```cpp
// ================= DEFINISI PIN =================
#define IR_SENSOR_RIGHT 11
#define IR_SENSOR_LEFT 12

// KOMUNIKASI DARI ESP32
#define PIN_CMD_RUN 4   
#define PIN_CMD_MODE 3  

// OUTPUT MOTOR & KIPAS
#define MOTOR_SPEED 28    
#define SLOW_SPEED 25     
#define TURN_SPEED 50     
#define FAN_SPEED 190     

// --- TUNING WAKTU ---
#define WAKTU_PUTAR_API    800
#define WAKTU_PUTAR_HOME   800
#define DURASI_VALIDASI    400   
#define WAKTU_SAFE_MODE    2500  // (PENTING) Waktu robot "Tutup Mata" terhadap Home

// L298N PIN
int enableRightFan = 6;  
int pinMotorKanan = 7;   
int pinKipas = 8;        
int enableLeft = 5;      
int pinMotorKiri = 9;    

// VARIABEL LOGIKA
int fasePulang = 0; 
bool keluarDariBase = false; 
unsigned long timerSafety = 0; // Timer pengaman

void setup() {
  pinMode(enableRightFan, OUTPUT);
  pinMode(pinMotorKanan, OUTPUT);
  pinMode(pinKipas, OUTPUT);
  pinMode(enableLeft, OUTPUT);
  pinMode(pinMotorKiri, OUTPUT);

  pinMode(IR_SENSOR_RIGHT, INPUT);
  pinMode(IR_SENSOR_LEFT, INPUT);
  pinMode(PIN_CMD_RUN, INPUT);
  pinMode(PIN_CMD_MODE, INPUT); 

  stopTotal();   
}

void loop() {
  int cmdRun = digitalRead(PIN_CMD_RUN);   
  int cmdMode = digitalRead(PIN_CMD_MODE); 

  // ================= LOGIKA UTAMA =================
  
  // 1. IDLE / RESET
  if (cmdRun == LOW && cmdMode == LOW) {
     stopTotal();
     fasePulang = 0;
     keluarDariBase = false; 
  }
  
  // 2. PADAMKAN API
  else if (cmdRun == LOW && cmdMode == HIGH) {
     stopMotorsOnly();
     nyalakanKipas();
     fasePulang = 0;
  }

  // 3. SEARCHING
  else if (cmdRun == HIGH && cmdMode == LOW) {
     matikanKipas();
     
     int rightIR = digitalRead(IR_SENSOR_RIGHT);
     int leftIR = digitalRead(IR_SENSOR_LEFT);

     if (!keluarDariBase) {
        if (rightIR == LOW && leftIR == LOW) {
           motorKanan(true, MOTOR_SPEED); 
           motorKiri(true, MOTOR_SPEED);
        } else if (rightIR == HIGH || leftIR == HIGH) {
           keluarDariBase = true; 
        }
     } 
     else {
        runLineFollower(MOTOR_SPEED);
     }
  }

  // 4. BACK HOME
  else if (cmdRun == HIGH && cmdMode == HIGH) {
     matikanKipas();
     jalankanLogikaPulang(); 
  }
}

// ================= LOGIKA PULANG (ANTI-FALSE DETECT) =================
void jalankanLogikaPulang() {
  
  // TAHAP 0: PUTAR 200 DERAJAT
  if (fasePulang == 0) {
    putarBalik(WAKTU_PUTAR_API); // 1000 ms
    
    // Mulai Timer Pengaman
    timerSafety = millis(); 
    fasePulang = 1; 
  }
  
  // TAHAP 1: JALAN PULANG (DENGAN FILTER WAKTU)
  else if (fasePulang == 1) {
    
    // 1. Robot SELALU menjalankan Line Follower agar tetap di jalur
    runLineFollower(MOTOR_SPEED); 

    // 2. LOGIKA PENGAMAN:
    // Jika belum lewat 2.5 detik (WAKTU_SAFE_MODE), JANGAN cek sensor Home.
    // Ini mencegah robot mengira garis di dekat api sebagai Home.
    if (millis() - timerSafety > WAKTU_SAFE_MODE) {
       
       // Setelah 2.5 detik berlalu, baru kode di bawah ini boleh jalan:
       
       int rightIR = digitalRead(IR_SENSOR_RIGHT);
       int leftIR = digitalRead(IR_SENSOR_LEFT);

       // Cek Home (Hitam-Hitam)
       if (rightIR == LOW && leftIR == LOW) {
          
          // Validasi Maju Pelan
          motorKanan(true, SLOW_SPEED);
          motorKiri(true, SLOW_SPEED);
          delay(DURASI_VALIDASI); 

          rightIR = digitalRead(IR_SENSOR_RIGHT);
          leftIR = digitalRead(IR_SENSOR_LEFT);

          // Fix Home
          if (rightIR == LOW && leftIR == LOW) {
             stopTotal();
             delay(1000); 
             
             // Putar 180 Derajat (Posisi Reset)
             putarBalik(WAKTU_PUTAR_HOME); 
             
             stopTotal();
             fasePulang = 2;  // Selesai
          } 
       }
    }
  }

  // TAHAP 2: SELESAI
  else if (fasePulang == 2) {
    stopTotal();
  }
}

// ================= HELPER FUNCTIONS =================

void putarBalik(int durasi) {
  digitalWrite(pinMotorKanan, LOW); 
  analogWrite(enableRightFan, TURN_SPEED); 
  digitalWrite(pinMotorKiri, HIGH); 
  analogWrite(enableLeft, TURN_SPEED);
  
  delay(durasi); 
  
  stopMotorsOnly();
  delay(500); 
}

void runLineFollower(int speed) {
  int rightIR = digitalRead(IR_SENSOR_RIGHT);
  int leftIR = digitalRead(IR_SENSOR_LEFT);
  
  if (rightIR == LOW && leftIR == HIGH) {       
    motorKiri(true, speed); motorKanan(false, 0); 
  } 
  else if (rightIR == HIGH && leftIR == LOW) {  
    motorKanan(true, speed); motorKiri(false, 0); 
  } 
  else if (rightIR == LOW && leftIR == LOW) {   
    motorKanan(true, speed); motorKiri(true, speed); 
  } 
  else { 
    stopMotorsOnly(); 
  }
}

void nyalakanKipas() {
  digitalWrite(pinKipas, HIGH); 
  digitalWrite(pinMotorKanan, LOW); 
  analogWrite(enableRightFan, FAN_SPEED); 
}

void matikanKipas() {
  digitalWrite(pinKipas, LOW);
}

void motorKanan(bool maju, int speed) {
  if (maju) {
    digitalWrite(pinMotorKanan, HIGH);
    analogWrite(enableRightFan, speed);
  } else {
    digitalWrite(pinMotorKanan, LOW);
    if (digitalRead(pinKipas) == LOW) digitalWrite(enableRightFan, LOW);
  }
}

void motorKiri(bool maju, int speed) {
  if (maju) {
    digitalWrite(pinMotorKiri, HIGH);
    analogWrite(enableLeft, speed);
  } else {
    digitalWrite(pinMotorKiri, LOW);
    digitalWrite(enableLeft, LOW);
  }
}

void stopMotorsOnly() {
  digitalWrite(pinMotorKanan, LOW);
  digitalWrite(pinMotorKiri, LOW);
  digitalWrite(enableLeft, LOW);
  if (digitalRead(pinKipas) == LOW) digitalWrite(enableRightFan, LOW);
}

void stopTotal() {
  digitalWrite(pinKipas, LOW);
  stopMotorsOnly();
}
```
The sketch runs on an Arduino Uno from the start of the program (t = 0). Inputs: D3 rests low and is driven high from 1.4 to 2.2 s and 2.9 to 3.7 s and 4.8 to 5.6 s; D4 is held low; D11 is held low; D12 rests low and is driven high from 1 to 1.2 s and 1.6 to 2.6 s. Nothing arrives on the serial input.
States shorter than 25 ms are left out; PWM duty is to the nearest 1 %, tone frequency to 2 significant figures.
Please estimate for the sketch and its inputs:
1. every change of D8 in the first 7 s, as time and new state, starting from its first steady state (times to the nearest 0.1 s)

0 s low; 1.4 s high; 2.2 s low; 2.9 s high; 3.7 s low; 4.8 s high; 5.6 s low
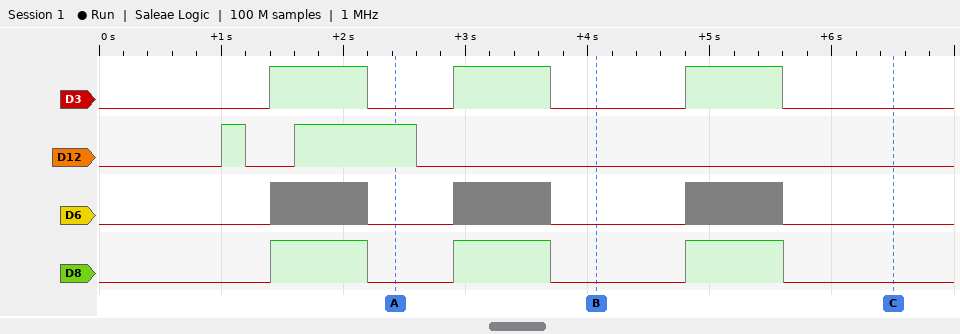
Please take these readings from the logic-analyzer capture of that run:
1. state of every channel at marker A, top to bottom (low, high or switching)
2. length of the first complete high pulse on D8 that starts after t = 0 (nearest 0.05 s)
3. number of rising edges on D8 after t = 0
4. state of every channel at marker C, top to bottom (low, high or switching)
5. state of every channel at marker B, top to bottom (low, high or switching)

D3 low, D12 high, D6 low, D8 low
0.80 s
3
D3 low, D12 low, D6 low, D8 low
D3 low, D12 low, D6 low, D8 low
